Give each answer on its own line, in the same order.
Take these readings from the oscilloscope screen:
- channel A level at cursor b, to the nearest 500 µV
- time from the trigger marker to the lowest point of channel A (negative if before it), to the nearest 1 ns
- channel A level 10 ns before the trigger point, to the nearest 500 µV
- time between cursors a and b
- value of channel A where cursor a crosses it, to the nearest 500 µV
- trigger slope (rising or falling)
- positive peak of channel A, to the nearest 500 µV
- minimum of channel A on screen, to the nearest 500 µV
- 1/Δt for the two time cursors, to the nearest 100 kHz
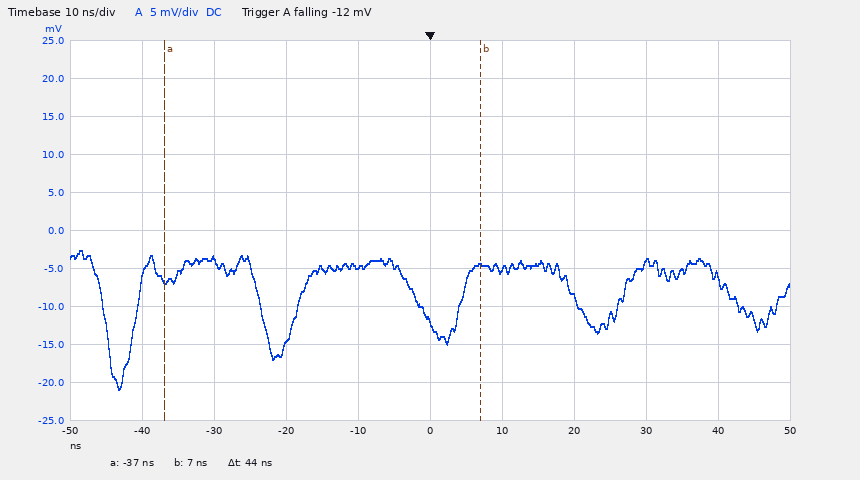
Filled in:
-4.5 mV
-43 ns
-5.0 mV
44 ns
-6.5 mV
falling
-2.5 mV
-21.0 mV
22.7 MHz
